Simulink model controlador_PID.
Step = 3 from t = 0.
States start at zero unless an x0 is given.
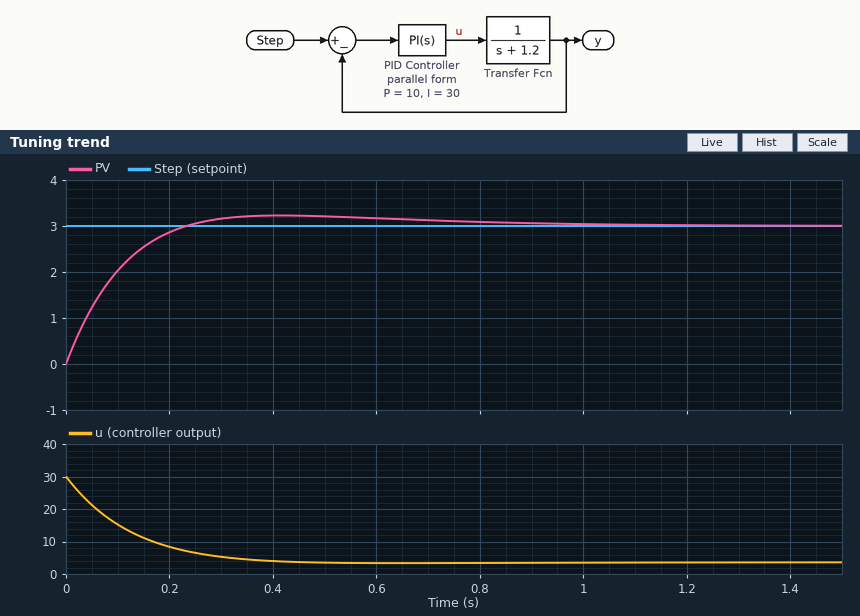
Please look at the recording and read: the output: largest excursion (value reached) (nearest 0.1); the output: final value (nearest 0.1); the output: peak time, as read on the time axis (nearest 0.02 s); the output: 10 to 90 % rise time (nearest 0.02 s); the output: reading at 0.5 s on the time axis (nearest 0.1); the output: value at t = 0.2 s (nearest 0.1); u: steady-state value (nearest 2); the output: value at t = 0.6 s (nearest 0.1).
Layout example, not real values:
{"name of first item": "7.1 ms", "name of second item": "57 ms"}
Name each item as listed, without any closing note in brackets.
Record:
{"the output: largest excursion (value reached)": "3.2", "the output: final value": "3.0", "the output: peak time, as read on the time axis": "0.42 s", "the output: 10 to 90 % rise time": "0.16 s", "the output: reading at 0.5 s on the time axis": "3.2", "the output: value at t = 0.2 s": "2.9", "u: steady-state value": "4", "the output: value at t = 0.6 s": "3.2"}
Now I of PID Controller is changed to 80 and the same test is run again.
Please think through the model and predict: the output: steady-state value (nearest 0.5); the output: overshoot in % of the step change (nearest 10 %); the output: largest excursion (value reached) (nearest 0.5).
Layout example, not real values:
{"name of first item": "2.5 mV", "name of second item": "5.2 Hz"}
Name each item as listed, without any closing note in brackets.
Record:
{"the output: steady-state value": "3.0", "the output: overshoot in % of the step change": "20 %", "the output: largest excursion (value reached)": "3.5"}
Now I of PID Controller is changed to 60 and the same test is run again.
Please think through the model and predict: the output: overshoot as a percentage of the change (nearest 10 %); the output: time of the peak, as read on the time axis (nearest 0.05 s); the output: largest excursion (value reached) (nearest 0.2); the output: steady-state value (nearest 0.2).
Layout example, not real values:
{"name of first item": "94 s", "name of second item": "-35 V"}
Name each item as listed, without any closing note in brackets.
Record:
{"the output: overshoot as a percentage of the change": "20 %", "the output: time of the peak, as read on the time axis": "0.30 s", "the output: largest excursion (value reached)": "3.4", "the output: steady-state value": "3.0"}
